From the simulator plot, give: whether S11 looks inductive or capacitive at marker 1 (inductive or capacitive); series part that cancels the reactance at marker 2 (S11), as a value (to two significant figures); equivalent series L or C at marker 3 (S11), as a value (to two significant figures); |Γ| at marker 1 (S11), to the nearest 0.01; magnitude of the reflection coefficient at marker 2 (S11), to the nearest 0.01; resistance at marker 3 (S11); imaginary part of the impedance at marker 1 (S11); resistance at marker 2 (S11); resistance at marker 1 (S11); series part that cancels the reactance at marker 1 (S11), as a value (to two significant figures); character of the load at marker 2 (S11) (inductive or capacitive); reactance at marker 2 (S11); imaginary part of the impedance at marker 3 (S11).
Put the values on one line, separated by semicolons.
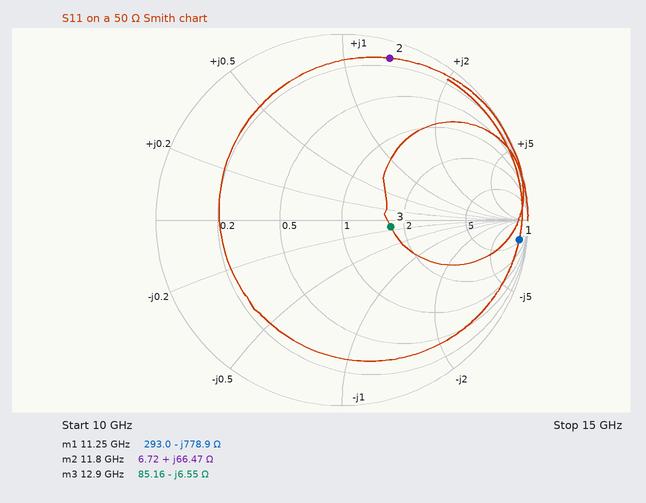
capacitive; 200 fF; 1.9 pF; 0.96; 0.91; 85.16 Ω; -778.9 Ω; 6.72 Ω; 293.0 Ω; 11 nH; inductive; +66.47 Ω; -6.55 Ω
